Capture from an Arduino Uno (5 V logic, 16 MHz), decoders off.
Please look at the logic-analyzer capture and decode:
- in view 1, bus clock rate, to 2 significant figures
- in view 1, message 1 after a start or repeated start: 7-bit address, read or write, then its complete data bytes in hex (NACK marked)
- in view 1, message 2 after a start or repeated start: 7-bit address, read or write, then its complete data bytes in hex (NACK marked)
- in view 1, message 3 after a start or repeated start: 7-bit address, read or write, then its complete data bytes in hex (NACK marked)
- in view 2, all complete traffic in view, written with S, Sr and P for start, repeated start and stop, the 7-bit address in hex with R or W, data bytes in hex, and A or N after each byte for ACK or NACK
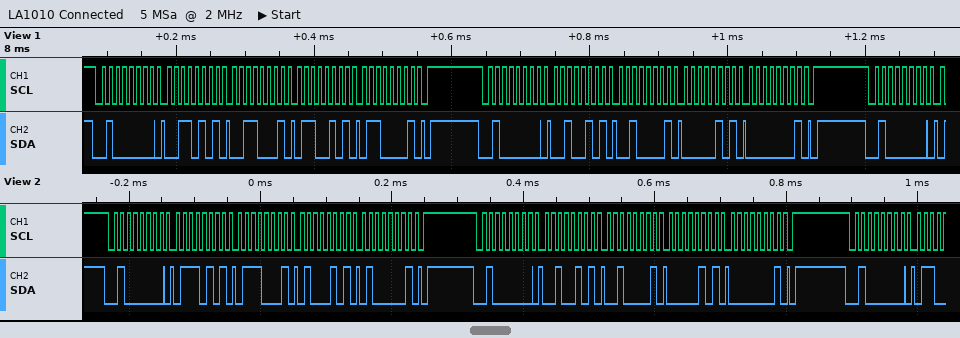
100 kHz
0x20 write: 35 31 65 61
0x20 write: 25 21 05 01
0x20 write
S 20W A 75 A 71 A 45 A 41 A P S 20W A 25 A 21 A 05 A 01 A P S 20W A
